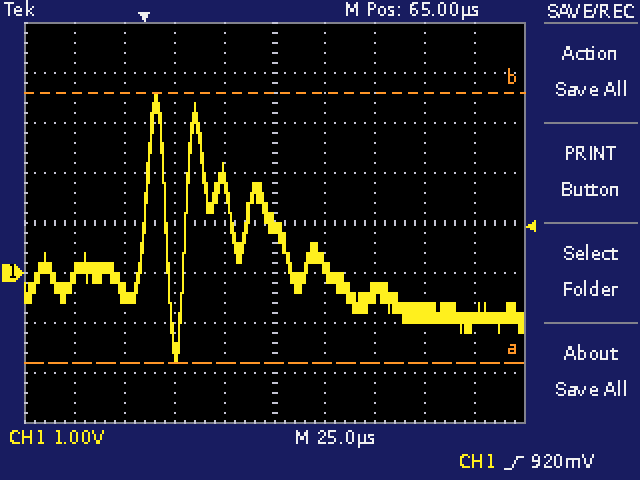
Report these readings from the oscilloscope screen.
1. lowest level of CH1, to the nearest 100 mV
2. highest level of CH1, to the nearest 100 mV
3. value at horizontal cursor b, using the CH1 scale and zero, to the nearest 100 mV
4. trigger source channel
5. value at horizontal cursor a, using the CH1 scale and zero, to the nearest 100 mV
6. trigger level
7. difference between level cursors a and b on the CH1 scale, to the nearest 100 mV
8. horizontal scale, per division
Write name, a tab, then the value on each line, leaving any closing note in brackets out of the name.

lowest level of CH1, to the nearest 100 mV	-1.8 V
highest level of CH1, to the nearest 100 mV	3.6 V
value at horizontal cursor b, using the CH1 scale and zero, to the nearest 100 mV	3.6 V
trigger source channel	CH1
value at horizontal cursor a, using the CH1 scale and zero, to the nearest 100 mV	-1.8 V
trigger level	920 mV
difference between level cursors a and b on the CH1 scale, to the nearest 100 mV	5.4 V
horizontal scale, per division	25 µs
